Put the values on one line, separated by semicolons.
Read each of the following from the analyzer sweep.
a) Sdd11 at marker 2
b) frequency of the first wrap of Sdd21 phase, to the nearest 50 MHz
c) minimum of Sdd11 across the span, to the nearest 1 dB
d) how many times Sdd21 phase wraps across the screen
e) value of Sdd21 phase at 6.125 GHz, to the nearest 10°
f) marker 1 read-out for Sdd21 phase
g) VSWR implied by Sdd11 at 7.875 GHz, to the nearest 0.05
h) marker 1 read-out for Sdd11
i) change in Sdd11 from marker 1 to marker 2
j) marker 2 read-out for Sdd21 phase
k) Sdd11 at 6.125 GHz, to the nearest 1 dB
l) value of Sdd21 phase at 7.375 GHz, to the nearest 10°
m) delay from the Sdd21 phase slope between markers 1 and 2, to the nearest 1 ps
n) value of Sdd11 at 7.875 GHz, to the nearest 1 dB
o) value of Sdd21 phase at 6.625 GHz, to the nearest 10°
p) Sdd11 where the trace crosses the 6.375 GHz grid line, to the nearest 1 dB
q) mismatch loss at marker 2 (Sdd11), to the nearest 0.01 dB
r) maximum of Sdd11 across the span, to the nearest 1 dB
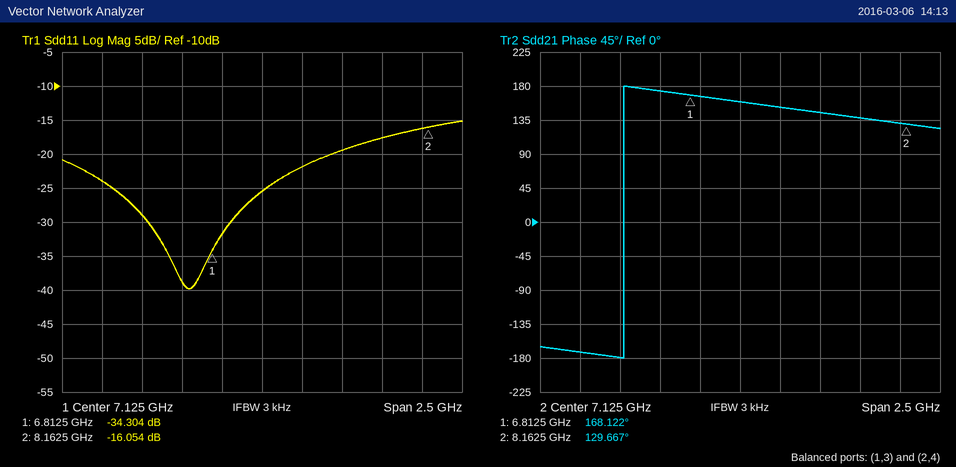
-16.054 dB; 6.40 GHz; -40 dB; 1; -170°; 168.122°; 1.30; -34.304 dB; 18.250 dB; 129.667°; -24 dB; 150°; 79 ps; -18 dB; 170°; -29 dB; 0.11 dB; -15 dB
